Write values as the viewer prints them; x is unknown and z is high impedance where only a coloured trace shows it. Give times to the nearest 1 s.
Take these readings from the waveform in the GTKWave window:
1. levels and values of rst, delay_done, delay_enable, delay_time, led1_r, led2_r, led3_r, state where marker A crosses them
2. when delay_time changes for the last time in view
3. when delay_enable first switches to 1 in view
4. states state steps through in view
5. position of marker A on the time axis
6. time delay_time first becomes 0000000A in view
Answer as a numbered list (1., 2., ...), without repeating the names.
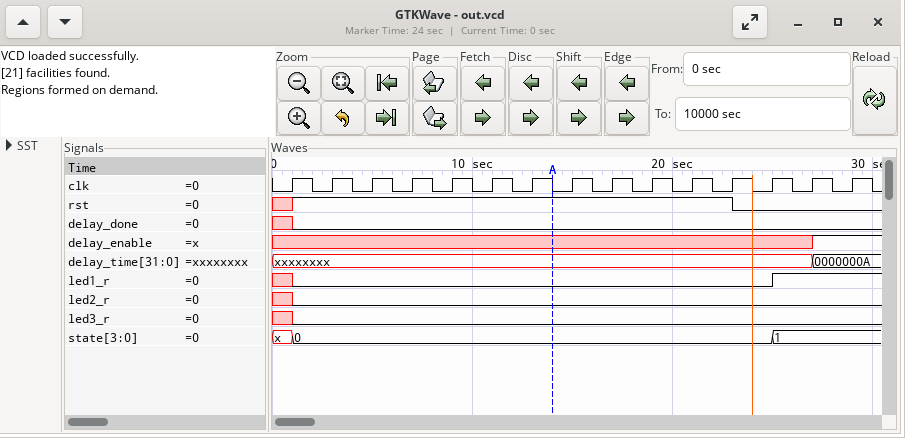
1. rst=1, delay_done=0, delay_enable=x, delay_time=xxxxxxxx, led1_r=0, led2_r=0, led3_r=0, state=0
2. 27 s
3. 27 s
4. x, 0, 1
5. 14 s
6. 27 s
